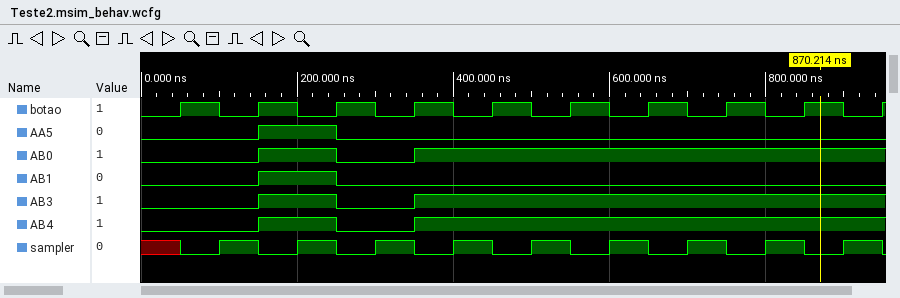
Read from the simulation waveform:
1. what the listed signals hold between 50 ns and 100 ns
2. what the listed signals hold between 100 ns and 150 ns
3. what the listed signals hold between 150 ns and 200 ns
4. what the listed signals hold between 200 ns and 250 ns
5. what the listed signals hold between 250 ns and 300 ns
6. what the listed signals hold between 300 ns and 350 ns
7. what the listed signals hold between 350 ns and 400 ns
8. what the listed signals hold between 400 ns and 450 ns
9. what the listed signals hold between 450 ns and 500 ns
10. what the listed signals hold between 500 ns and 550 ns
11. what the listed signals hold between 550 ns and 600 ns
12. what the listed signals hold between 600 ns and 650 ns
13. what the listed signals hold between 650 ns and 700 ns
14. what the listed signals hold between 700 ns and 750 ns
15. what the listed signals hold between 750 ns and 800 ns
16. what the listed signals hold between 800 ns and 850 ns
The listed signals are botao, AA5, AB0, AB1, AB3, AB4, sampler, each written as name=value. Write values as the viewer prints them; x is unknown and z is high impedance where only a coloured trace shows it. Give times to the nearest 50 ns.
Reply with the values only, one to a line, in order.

botao=1, AA5=0, AB0=0, AB1=0, AB3=0, AB4=0, sampler=0
botao=0, AA5=0, AB0=0, AB1=0, AB3=0, AB4=0, sampler=1
botao=1, AA5=1, AB0=1, AB1=1, AB3=1, AB4=1, sampler=0
botao=0, AA5=1, AB0=1, AB1=1, AB3=1, AB4=1, sampler=1
botao=1, AA5=0, AB0=0, AB1=0, AB3=0, AB4=0, sampler=0
botao=0, AA5=0, AB0=0, AB1=0, AB3=0, AB4=0, sampler=1
botao=1, AA5=0, AB0=1, AB1=0, AB3=1, AB4=1, sampler=0
botao=0, AA5=0, AB0=1, AB1=0, AB3=1, AB4=1, sampler=1
botao=1, AA5=0, AB0=1, AB1=0, AB3=1, AB4=1, sampler=0
botao=0, AA5=0, AB0=1, AB1=0, AB3=1, AB4=1, sampler=1
botao=1, AA5=0, AB0=1, AB1=0, AB3=1, AB4=1, sampler=0
botao=0, AA5=0, AB0=1, AB1=0, AB3=1, AB4=1, sampler=1
botao=1, AA5=0, AB0=1, AB1=0, AB3=1, AB4=1, sampler=0
botao=0, AA5=0, AB0=1, AB1=0, AB3=1, AB4=1, sampler=1
botao=1, AA5=0, AB0=1, AB1=0, AB3=1, AB4=1, sampler=0
botao=0, AA5=0, AB0=1, AB1=0, AB3=1, AB4=1, sampler=1
